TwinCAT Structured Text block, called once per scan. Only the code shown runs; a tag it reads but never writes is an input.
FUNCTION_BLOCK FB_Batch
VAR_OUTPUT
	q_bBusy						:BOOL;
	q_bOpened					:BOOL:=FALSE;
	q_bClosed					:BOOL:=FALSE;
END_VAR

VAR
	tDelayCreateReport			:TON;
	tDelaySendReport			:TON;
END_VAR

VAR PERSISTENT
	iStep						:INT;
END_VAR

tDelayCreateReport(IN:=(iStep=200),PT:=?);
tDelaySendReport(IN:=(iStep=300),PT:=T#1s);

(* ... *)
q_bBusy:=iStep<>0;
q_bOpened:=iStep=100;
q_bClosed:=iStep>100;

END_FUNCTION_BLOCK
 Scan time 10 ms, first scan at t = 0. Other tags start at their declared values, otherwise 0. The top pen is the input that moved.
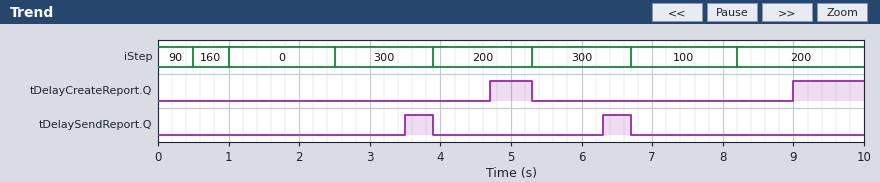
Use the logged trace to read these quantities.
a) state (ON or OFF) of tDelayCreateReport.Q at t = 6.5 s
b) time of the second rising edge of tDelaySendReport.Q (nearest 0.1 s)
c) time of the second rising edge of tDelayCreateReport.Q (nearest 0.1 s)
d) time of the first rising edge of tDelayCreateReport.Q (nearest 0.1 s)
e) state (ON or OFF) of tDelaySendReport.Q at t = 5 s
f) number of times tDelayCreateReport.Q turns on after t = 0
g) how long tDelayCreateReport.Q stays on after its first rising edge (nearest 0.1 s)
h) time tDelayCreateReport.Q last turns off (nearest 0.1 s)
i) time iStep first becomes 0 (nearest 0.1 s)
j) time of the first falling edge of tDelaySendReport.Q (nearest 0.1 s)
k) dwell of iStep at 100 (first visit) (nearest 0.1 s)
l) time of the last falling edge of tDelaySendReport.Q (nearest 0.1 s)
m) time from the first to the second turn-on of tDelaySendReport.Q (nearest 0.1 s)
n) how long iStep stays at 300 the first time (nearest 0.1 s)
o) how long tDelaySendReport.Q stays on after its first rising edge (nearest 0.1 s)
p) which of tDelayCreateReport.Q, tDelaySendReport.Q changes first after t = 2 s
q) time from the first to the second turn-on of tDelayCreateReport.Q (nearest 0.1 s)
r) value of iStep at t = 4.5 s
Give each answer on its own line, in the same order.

OFF
6.3 s
9.0 s
4.7 s
OFF
2
0.6 s
5.3 s
1.0 s
3.9 s
1.5 s
6.7 s
2.8 s
1.4 s
0.4 s
tDelaySendReport.Q
4.3 s
200
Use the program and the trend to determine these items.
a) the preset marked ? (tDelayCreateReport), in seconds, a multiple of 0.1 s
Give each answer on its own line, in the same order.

0.8 s
